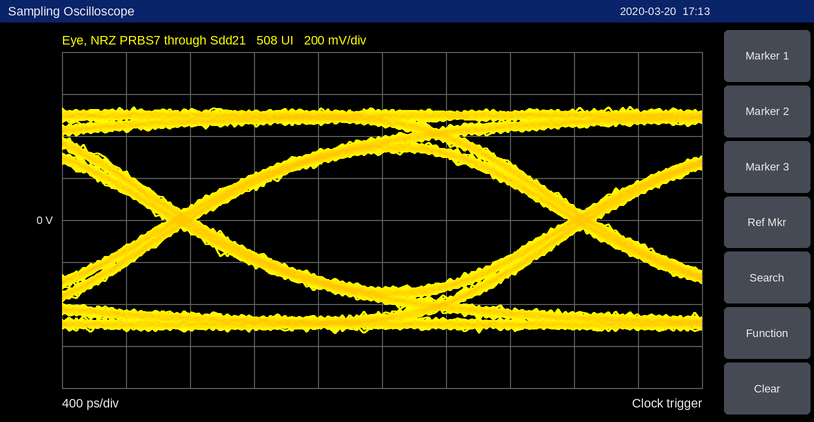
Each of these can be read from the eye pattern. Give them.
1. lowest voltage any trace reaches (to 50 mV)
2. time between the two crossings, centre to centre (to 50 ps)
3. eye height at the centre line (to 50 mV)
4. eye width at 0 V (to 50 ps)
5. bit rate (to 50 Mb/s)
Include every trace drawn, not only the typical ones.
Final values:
-550 mV
2.50 ns
650 mV
2.35 ns
400 Mb/s
